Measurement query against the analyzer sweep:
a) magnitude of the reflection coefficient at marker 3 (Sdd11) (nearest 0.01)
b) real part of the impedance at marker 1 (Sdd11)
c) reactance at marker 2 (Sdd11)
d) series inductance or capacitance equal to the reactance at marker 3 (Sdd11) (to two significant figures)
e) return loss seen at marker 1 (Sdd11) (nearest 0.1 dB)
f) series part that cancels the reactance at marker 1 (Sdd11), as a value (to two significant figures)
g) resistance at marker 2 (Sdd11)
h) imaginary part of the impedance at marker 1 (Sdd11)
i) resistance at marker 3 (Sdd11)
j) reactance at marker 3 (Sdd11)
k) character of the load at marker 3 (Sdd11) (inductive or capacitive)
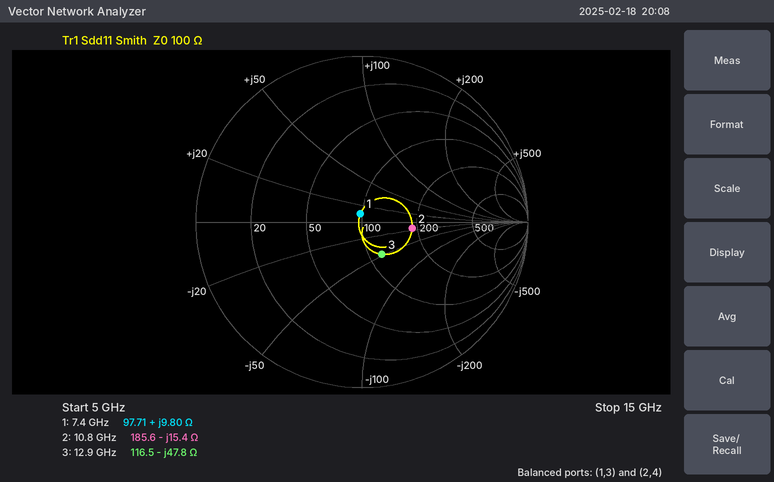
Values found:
0.23
97.71 Ω
-15.4 Ω
260 fF
25.9 dB
2.2 pF
185.6 Ω
+9.80 Ω
116.5 Ω
-47.8 Ω
capacitive
